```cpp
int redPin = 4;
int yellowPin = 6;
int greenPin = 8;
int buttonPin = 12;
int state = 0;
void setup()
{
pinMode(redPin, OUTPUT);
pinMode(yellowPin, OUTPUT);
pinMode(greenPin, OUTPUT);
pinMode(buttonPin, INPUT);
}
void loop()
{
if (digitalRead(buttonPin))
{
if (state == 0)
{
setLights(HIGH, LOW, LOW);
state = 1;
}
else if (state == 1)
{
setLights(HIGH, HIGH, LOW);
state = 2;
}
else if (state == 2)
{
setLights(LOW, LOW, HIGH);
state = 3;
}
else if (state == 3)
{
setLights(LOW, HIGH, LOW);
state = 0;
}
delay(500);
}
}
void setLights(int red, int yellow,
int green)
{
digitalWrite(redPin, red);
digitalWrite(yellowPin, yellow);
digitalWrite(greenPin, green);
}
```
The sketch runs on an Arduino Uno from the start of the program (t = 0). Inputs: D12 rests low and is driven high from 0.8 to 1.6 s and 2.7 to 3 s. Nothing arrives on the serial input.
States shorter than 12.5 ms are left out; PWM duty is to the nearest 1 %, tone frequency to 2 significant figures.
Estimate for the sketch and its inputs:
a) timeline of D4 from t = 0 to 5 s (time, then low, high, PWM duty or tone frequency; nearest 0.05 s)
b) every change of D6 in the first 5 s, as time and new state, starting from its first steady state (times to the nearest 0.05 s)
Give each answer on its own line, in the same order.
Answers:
0 s low; 0.8 s high; 2.7 s low
0 s low; 1.3 s high; 2.7 s low
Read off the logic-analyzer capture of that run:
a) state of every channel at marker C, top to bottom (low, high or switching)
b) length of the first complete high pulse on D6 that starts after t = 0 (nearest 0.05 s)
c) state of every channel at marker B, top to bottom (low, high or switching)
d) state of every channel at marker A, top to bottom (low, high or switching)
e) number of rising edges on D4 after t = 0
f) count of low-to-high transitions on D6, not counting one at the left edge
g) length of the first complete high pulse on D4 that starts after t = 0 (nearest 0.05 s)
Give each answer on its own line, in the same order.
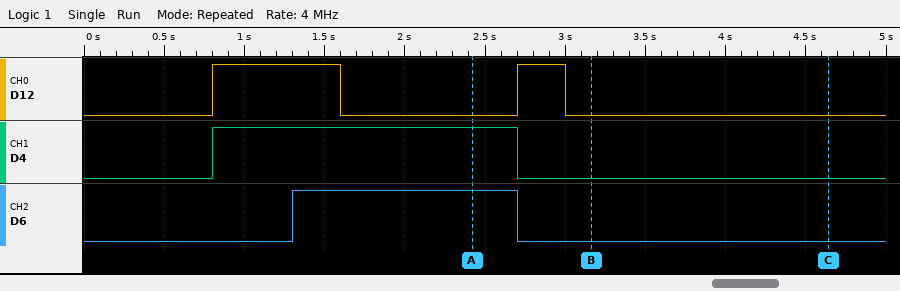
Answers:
D12 low, D4 low, D6 low
1.40 s
D12 low, D4 low, D6 low
D12 low, D4 high, D6 high
1
1
1.90 s
